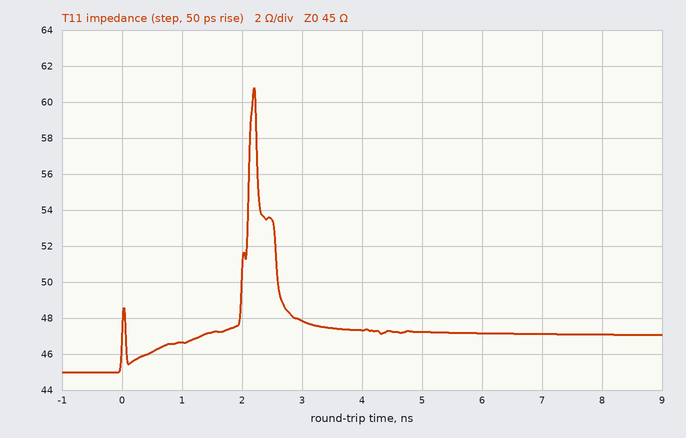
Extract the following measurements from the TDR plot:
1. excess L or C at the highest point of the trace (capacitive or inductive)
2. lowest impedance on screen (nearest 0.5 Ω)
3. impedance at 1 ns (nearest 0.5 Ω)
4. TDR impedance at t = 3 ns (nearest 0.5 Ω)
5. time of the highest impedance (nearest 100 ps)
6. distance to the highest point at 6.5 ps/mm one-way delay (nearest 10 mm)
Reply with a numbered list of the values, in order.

1. inductive
2. 45.0 Ω
3. 46.5 Ω
4. 48.0 Ω
5. 2.2 ns
6. 170 mm
